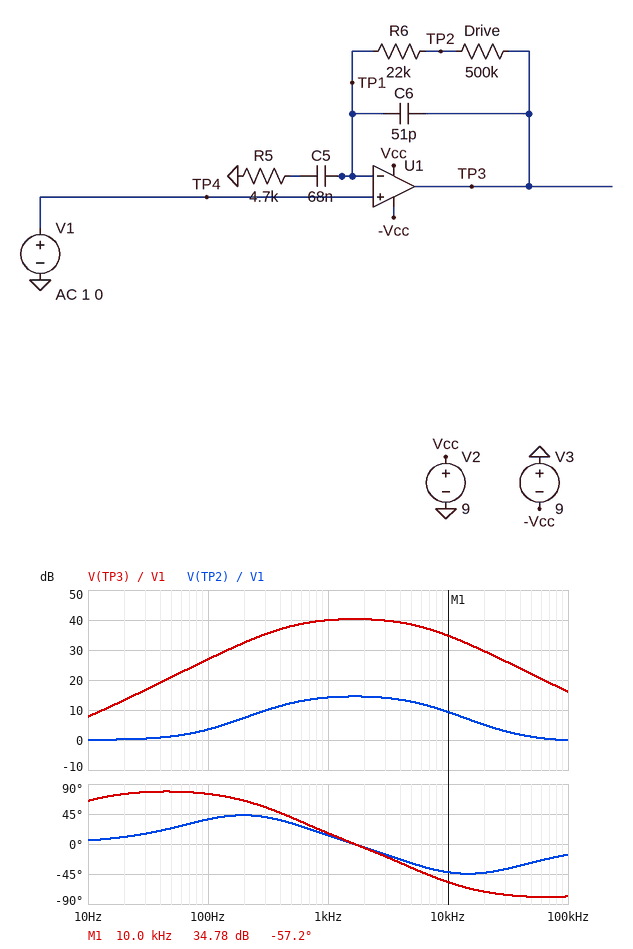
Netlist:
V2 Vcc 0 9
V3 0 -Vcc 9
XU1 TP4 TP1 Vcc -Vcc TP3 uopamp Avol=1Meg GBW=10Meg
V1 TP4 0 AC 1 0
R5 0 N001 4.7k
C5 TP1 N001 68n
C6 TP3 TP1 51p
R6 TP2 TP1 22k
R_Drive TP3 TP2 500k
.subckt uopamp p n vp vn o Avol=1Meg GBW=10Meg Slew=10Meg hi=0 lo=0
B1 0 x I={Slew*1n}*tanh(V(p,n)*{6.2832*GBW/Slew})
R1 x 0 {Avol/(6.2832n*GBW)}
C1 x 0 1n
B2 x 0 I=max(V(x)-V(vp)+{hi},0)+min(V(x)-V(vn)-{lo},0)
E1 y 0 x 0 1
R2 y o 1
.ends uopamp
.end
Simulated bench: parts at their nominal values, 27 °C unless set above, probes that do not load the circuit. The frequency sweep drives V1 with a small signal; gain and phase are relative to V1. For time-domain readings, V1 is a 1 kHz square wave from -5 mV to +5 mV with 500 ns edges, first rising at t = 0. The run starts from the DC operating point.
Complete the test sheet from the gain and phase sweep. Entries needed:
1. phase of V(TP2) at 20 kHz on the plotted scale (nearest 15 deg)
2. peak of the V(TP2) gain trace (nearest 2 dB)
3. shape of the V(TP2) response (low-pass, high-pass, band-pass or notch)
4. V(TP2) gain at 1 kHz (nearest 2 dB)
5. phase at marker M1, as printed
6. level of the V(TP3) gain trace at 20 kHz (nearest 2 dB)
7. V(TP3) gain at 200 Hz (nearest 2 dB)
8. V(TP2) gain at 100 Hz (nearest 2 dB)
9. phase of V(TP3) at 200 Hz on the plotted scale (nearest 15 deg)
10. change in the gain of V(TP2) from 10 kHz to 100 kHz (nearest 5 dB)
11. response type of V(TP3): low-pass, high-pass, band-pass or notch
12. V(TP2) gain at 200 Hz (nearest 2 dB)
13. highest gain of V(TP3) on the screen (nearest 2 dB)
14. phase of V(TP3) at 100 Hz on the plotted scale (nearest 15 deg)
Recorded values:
-45 deg
14 dB
band-pass
14 dB
-57.2 deg
30 dB
32 dB
4 dB
60 deg
-10 dB
band-pass
8 dB
40 dB
75 deg
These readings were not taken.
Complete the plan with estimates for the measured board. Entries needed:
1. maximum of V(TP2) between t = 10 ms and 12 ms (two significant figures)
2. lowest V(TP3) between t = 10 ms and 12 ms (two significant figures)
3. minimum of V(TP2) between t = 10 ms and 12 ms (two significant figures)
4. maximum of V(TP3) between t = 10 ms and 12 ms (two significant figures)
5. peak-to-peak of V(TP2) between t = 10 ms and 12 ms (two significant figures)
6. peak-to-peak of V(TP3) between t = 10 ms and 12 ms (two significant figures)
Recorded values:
35 mV
-720 mV
-35 mV
720 mV
70 mV
1.4 V
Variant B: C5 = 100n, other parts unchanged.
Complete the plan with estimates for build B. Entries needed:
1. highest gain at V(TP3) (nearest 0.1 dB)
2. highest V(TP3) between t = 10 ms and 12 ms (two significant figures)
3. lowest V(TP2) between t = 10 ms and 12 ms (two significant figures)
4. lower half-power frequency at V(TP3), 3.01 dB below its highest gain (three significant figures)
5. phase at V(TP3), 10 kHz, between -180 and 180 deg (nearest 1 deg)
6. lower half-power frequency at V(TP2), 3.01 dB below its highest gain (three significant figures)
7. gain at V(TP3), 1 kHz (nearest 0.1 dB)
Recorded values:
40.5 dB
680 mV
-34 mV
305 Hz
-58 deg
295 Hz
40.4 dB
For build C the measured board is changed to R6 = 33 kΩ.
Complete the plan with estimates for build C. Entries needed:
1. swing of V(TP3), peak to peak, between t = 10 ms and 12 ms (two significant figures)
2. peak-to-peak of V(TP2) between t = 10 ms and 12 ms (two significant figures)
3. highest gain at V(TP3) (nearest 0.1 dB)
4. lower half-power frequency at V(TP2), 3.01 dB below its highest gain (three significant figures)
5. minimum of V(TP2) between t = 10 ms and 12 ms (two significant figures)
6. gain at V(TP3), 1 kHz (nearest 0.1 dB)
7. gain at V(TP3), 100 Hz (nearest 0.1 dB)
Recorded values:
1.5 V
100 mV
40.5 dB
421 Hz
-50 mV
40.1 dB
27.1 dB
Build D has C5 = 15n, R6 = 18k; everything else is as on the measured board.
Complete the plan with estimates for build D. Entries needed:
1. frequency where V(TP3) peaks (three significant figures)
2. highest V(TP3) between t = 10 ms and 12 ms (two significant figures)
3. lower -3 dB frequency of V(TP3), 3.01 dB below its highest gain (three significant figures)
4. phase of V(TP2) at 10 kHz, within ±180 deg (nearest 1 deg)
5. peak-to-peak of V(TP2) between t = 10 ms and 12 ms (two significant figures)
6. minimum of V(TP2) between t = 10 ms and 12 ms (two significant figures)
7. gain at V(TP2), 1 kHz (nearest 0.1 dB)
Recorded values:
3.57 kHz
610 mV
1.39 kHz
-33 deg
52 mV
-26 mV
7.0 dB
